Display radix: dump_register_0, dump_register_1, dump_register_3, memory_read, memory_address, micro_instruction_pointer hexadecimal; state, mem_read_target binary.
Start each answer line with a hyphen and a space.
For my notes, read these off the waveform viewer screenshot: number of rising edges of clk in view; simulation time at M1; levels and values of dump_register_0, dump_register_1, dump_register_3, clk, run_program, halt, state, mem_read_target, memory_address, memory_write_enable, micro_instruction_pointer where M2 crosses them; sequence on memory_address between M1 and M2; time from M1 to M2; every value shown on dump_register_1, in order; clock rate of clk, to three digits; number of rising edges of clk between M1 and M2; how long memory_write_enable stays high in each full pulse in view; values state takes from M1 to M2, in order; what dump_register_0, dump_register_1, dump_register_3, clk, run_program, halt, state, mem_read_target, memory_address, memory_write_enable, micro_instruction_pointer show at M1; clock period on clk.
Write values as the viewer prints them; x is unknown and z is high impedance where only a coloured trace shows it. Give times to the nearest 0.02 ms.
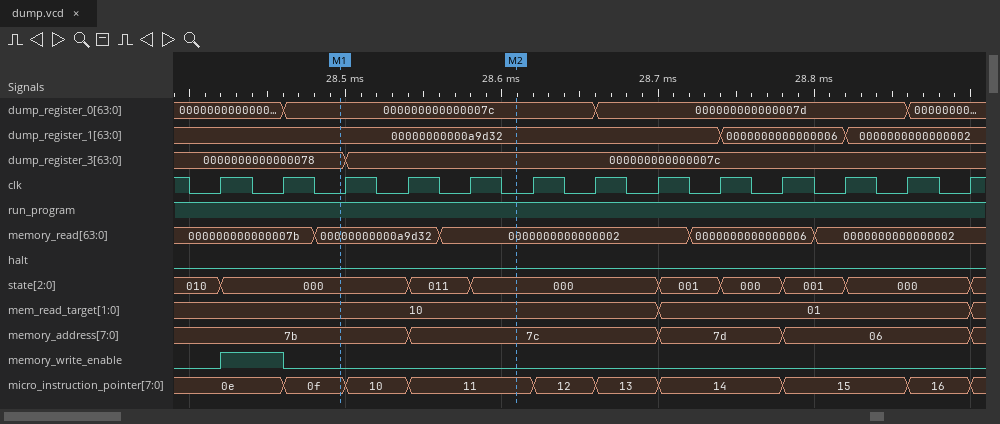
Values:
- 13
- 28.5 ms
- dump_register_0=000000000000007c, dump_register_1=00000000000a9d32, dump_register_3=000000000000007c, clk=0, run_program=1, halt=0, state=000, mem_read_target=10, memory_address=7c, memory_write_enable=0, micro_instruction_pointer=11
- 7b, 7c
- 0.12 ms
- 00000000000a9d32, 0000000000000006, 0000000000000002
- 25.0 kHz
- 3
- 0.04 ms
- 000, 011, 000
- dump_register_0=000000000000007c, dump_register_1=00000000000a9d32, dump_register_3=0000000000000078, clk=0, run_program=1, halt=0, state=000, mem_read_target=10, memory_address=7b, memory_write_enable=0, micro_instruction_pointer=0f
- 0.04 ms
